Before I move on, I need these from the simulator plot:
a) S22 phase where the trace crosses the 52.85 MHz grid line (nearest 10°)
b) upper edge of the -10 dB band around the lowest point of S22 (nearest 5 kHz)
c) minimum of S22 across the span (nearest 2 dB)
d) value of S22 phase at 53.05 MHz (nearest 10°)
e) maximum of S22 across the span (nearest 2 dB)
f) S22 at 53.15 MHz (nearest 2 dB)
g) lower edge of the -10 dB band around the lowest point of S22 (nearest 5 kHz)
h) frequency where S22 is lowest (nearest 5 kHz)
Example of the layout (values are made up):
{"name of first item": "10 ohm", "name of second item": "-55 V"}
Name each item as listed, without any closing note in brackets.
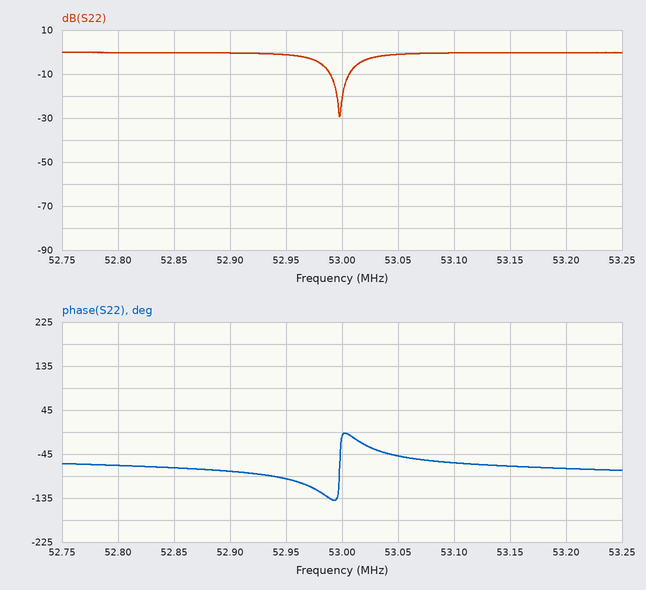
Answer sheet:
{"S22 phase where the trace crosses the 52.85 MHz grid line": "-70°", "upper edge of the -10 dB band around the lowest point of S22": "53.005 MHz", "minimum of S22 across the span": "-30 dB", "value of S22 phase at 53.05 MHz": "-50°", "maximum of S22 across the span": "0 dB", "S22 at 53.15 MHz": "0 dB", "lower edge of the -10 dB band around the lowest point of S22": "52.990 MHz", "frequency where S22 is lowest": "53.000 MHz"}
